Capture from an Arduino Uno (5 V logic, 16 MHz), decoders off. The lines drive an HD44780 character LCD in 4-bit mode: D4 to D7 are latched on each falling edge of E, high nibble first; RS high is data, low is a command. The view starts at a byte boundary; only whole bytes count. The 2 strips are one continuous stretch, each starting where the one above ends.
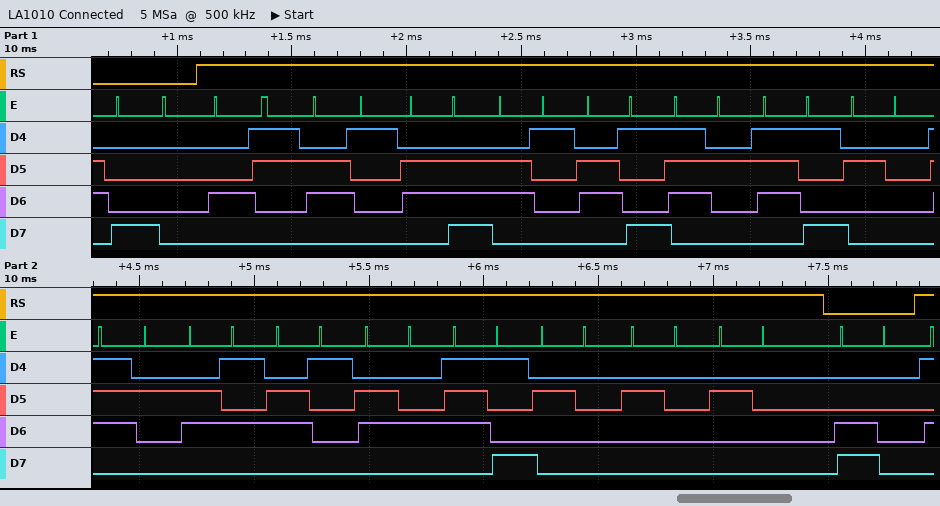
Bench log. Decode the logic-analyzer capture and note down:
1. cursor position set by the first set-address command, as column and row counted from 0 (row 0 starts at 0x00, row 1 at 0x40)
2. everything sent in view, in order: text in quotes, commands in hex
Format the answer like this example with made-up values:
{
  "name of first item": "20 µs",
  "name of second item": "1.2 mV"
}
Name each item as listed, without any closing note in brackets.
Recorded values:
{
  "cursor position set by the first set-address command, as column and row counted from 0": "column 0, row 0",
  "everything sent in view, in order: text in quotes, commands in hex": "0x80 \"Canairy ready   \" 0xC0"
}
